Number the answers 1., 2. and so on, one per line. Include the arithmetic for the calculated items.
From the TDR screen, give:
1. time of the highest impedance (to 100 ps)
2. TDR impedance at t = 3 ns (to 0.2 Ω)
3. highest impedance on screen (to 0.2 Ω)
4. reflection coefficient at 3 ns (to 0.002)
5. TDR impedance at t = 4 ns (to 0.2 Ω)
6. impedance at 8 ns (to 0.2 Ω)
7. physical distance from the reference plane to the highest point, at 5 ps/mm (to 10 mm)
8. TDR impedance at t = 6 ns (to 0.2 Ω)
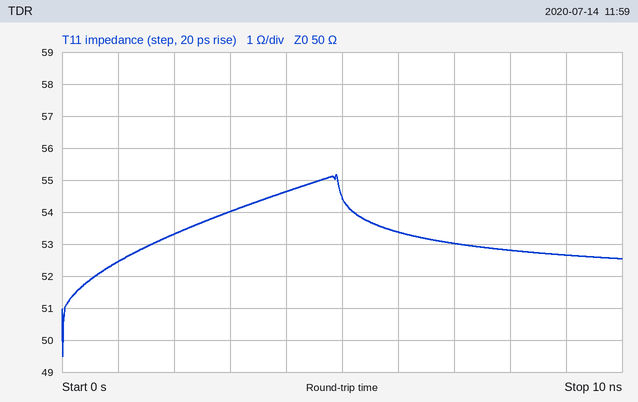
1. 4.9 ns
2. 54.0 Ω
3. 55.2 Ω
4. (54 − 50)/(54 + 50) ≈ +0.038
5. 54.6 Ω
6. 52.8 Ω
7. 4.9 ns / 2 / 5 ps/mm ≈ 490 mm
8. 53.4 Ω
